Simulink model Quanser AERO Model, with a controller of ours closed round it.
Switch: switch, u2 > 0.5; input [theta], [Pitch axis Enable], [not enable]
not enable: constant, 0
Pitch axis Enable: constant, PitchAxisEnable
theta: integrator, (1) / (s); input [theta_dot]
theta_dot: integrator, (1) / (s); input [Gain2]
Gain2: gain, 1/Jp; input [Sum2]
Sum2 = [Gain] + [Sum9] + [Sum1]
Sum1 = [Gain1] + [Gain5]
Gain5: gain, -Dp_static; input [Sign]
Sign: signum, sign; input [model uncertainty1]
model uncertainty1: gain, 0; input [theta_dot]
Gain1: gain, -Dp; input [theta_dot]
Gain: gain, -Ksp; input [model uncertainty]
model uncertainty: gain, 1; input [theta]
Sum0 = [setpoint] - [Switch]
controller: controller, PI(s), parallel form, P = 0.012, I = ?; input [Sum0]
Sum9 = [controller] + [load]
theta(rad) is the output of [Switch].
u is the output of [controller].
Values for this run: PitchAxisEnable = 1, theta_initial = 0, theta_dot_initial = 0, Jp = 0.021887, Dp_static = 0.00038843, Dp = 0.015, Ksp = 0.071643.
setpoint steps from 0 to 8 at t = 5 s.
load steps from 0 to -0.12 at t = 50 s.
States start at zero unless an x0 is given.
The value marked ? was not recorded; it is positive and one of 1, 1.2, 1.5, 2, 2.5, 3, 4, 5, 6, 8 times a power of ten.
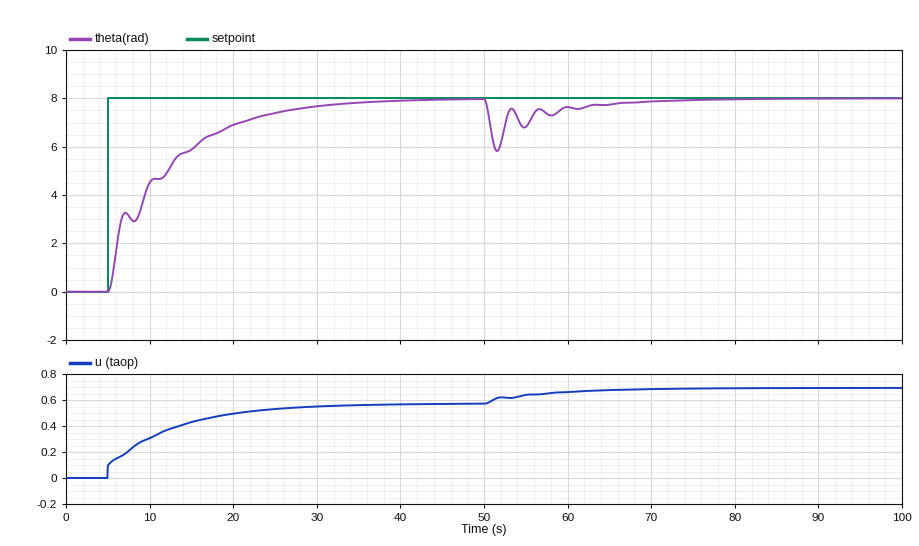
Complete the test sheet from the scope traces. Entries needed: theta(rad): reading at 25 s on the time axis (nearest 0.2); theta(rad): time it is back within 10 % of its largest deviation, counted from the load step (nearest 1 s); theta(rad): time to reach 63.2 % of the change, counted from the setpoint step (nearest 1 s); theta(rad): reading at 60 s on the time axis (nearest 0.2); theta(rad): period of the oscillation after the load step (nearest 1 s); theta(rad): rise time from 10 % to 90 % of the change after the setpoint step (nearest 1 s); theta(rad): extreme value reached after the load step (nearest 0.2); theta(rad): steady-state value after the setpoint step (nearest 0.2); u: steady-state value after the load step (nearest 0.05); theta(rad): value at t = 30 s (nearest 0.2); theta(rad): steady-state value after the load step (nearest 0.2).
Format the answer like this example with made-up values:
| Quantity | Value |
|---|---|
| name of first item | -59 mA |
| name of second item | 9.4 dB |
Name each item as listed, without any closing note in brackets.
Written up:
| Quantity | Value |
|---|---|
| theta(rad): reading at 25 s on the time axis | 7.4 |
| theta(rad): time it is back within 10 % of its largest deviation, counted from the load step | 16 s |
| theta(rad): time to reach 63.2 % of the change, counted from the setpoint step | 7 s |
| theta(rad): reading at 60 s on the time axis | 7.6 |
| theta(rad): period of the oscillation after the load step | 3 s |
| theta(rad): rise time from 10 % to 90 % of the change after the setpoint step | 17 s |
| theta(rad): extreme value reached after the load step | 5.8 |
| theta(rad): steady-state value after the setpoint step | 8.0 |
| u: steady-state value after the load step | 0.70 |
| theta(rad): value at t = 30 s | 7.6 |
| theta(rad): steady-state value after the load step | 8.0 |
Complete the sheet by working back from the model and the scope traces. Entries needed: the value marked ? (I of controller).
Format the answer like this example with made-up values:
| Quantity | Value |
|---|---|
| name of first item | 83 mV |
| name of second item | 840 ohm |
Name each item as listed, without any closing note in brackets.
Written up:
| Quantity | Value |
|---|---|
| the value marked ? | 0.01 |
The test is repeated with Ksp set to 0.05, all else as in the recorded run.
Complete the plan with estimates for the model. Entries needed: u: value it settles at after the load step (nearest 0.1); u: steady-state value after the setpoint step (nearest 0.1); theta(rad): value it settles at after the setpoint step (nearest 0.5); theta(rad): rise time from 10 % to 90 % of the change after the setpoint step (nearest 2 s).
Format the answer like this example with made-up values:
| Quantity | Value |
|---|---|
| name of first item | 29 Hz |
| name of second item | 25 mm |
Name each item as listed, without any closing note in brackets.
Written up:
| Quantity | Value |
|---|---|
| u: value it settles at after the load step | 0.5 |
| u: steady-state value after the setpoint step | 0.4 |
| theta(rad): value it settles at after the setpoint step | 8.0 |
| theta(rad): rise time from 10 % to 90 % of the change after the setpoint step | 12 s |
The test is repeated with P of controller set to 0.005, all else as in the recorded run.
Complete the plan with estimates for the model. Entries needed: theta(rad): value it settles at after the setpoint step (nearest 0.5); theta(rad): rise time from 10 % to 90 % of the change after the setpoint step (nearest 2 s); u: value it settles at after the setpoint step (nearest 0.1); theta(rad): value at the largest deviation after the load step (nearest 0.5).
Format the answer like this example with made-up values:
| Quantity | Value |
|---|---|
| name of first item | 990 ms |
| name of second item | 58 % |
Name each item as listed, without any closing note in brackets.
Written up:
| Quantity | Value |
|---|---|
| theta(rad): value it settles at after the setpoint step | 8.0 |
| theta(rad): rise time from 10 % to 90 % of the change after the setpoint step | 16 s |
| u: value it settles at after the setpoint step | 0.6 |
| theta(rad): value at the largest deviation after the load step | 5.5 |
